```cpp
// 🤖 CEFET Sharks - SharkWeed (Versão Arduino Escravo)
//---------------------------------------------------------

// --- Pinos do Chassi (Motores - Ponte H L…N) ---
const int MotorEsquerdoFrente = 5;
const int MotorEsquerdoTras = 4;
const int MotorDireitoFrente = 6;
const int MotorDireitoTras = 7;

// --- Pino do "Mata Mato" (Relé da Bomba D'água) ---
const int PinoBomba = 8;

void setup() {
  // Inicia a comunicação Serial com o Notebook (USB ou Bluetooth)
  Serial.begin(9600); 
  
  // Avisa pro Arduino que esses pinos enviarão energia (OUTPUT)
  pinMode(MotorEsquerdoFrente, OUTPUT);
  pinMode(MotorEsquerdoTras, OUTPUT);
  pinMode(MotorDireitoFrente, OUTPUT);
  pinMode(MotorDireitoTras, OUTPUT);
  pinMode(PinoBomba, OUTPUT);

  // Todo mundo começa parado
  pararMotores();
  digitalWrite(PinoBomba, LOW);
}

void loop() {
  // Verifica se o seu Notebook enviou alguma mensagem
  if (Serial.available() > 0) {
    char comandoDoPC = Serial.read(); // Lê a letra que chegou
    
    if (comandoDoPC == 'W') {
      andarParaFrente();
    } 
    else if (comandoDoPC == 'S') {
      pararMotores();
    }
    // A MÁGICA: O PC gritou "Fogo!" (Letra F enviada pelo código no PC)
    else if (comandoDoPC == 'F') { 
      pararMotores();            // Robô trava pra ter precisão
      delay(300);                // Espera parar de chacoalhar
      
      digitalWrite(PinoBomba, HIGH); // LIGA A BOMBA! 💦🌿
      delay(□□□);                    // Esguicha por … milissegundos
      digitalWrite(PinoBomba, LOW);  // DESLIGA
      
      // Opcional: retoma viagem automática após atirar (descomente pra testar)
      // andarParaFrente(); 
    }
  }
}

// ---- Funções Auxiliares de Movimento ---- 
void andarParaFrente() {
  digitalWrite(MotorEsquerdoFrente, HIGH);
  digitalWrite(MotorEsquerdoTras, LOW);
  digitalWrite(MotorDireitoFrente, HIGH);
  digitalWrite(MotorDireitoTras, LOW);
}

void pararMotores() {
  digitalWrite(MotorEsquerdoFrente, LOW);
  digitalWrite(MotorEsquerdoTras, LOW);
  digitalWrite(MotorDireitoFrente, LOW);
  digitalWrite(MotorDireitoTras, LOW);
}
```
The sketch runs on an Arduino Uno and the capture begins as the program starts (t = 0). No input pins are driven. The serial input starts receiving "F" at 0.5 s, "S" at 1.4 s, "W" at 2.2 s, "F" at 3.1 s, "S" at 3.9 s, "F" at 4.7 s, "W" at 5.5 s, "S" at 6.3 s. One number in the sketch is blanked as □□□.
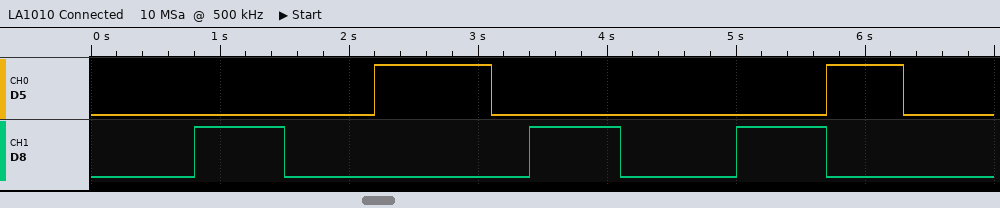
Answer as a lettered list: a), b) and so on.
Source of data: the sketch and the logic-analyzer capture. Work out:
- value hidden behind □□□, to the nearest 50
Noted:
a) 700
